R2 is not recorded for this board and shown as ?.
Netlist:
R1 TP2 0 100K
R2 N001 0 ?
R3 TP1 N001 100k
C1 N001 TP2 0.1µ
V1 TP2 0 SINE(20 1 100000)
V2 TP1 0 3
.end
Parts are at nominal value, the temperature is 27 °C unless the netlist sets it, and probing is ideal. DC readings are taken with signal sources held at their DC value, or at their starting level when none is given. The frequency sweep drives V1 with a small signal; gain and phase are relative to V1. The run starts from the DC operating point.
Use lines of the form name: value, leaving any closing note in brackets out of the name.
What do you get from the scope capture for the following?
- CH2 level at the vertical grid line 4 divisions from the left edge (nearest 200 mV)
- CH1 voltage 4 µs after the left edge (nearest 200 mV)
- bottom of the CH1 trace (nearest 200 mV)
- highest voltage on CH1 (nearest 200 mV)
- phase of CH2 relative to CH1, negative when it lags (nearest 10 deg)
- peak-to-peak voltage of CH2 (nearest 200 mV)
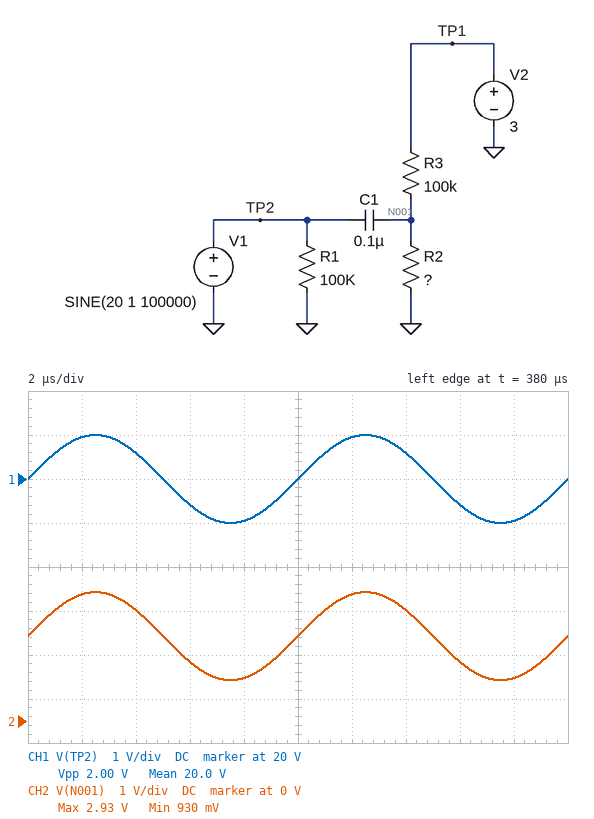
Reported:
CH2 level at the vertical grid line 4 divisions from the left edge: 1.0 V
CH1 voltage 4 µs after the left edge: 20.6 V
bottom of the CH1 trace: 19.0 V
highest voltage on CH1: 21.0 V
phase of CH2 relative to CH1, negative when it lags: 0 deg
peak-to-peak voltage of CH2: 2.0 V
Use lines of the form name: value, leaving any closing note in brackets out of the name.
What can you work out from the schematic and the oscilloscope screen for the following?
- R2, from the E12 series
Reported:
R2, from the E12 series: 180 kΩ
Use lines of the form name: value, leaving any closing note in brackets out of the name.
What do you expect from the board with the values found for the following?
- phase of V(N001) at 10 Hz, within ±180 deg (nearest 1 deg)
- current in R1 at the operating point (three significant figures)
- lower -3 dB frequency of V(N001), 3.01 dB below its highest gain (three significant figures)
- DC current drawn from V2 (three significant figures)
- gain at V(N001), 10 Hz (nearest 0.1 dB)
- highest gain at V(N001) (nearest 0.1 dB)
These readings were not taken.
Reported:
phase of V(N001) at 10 Hz, within ±180 deg: 68 deg
current in R1 at the operating point: 200 µA
lower -3 dB frequency of V(N001), 3.01 dB below its highest gain: 24.8 Hz
DC current drawn from V2: 10.7 µA
gain at V(N001), 10 Hz: -8.5 dB
highest gain at V(N001): 0 dB
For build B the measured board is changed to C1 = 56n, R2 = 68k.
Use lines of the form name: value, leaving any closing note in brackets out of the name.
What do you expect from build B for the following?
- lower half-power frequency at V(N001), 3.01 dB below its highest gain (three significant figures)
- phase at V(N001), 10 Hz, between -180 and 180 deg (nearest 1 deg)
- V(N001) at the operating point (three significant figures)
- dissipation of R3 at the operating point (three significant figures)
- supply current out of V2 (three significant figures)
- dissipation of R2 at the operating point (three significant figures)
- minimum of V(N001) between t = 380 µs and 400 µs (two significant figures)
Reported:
lower half-power frequency at V(N001), 3.01 dB below its highest gain: 70.2 Hz
phase at V(N001), 10 Hz, between -180 and 180 deg: 82 deg
V(N001) at the operating point: 1.21 V
dissipation of R3 at the operating point: 31.9 µW
supply current out of V2: 17.9 µA
dissipation of R2 at the operating point: 21.7 µW
minimum of V(N001) between t = 380 µs and 400 µs: 210 mV
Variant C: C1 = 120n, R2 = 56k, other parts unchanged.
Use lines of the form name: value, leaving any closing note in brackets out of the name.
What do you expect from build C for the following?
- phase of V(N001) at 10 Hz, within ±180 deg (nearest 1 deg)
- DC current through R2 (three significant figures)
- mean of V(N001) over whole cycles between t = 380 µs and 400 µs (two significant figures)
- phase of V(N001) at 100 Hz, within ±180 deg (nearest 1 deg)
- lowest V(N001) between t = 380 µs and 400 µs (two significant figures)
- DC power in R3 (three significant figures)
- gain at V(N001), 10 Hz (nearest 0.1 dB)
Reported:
phase of V(N001) at 10 Hz, within ±180 deg: 75 deg
DC current through R2: 19.2 µA
mean of V(N001) over whole cycles between t = 380 µs and 400 µs: 1.1 V
phase of V(N001) at 100 Hz, within ±180 deg: 20 deg
lowest V(N001) between t = 380 µs and 400 µs: 77 mV
DC power in R3: 37.0 µW
gain at V(N001), 10 Hz: -11.7 dB
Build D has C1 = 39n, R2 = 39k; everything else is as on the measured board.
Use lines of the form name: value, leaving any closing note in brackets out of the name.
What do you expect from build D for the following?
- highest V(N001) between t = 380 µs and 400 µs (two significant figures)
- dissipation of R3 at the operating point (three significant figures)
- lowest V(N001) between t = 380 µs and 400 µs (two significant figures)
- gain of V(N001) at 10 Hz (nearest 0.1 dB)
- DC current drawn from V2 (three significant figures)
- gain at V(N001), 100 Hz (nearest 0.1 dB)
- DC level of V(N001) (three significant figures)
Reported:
highest V(N001) between t = 380 µs and 400 µs: 1.8 V
dissipation of R3 at the operating point: 46.6 µW
lowest V(N001) between t = 380 µs and 400 µs: -160 mV
gain of V(N001) at 10 Hz: -23.3 dB
DC current drawn from V2: 21.6 µA
gain at V(N001), 100 Hz: -4.9 dB
DC level of V(N001): 842 mV
